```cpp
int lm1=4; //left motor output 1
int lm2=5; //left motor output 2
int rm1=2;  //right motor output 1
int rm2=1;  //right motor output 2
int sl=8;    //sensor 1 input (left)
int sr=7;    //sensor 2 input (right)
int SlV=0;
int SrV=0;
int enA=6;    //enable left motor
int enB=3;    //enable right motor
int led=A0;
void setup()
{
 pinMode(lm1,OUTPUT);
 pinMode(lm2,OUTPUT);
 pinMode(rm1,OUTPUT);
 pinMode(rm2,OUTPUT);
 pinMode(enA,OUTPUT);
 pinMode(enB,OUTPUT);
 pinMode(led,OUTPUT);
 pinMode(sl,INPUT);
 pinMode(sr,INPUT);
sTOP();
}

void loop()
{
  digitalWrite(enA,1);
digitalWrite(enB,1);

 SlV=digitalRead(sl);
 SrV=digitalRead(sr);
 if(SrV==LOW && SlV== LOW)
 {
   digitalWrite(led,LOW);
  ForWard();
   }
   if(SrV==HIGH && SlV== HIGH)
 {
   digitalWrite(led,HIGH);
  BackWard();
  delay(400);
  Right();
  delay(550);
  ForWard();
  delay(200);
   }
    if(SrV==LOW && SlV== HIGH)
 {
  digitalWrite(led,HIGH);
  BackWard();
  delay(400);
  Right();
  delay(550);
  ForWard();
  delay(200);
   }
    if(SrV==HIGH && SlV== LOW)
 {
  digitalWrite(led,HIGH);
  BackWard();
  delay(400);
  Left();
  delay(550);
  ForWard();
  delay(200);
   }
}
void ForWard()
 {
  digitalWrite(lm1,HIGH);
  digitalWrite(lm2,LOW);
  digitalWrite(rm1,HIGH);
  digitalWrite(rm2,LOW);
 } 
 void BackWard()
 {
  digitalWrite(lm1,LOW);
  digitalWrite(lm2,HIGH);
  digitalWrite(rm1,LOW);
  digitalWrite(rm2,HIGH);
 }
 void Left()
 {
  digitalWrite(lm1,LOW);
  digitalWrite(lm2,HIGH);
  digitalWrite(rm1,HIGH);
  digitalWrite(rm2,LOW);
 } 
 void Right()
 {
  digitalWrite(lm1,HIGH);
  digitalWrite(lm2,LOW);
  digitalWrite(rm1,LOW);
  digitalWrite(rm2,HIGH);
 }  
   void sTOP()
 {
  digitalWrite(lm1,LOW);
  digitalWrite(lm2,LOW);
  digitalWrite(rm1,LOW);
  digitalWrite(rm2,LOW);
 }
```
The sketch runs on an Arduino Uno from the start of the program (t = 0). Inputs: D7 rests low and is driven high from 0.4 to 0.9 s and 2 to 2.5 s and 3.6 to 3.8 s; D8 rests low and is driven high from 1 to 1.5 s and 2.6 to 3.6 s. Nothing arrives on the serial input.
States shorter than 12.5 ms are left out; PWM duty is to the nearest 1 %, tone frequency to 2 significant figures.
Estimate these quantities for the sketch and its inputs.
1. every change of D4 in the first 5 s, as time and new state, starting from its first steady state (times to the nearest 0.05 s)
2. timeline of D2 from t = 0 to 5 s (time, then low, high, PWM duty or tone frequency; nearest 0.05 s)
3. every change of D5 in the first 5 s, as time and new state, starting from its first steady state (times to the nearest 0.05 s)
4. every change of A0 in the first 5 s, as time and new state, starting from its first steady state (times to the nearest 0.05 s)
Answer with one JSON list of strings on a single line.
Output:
["0 s high; 0.4 s low; 1.35 s high; 2 s low; 2.95 s high; 3.15 s low; 3.55 s high", "0 s high; 0.4 s low; 0.8 s high; 2 s low; 2.4 s high; 3.15 s low; 4.1 s high", "0 s low; 0.4 s high; 1.35 s low; 2 s high; 2.95 s low; 3.15 s high; 3.55 s low", "0 s low; 0.4 s high; 1.55 s low; 2 s high; 4.3 s low"]
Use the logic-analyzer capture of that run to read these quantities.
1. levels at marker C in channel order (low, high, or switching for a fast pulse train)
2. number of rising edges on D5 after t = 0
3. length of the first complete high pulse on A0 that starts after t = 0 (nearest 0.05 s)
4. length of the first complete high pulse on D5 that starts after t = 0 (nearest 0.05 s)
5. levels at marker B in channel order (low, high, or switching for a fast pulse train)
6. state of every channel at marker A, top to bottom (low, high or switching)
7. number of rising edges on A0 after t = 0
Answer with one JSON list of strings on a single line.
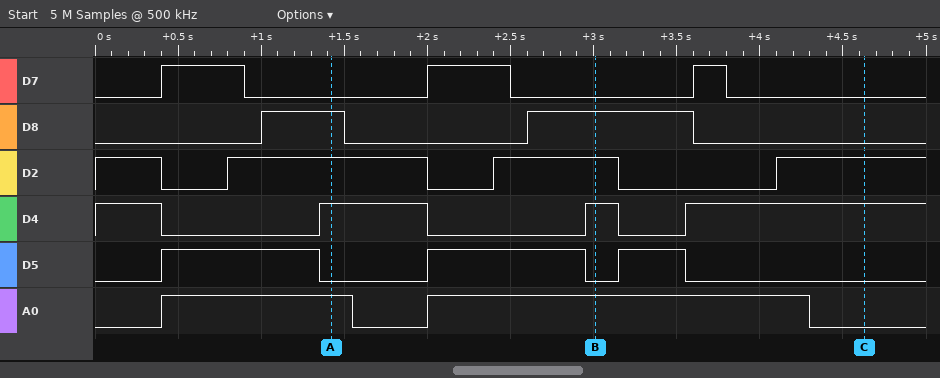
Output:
["D7 low, D8 low, D2 high, D4 high, D5 low, A0 low", "3", "1.15 s", "0.95 s", "D7 low, D8 high, D2 high, D4 high, D5 low, A0 high", "D7 low, D8 high, D2 high, D4 high, D5 low, A0 high", "2"]
